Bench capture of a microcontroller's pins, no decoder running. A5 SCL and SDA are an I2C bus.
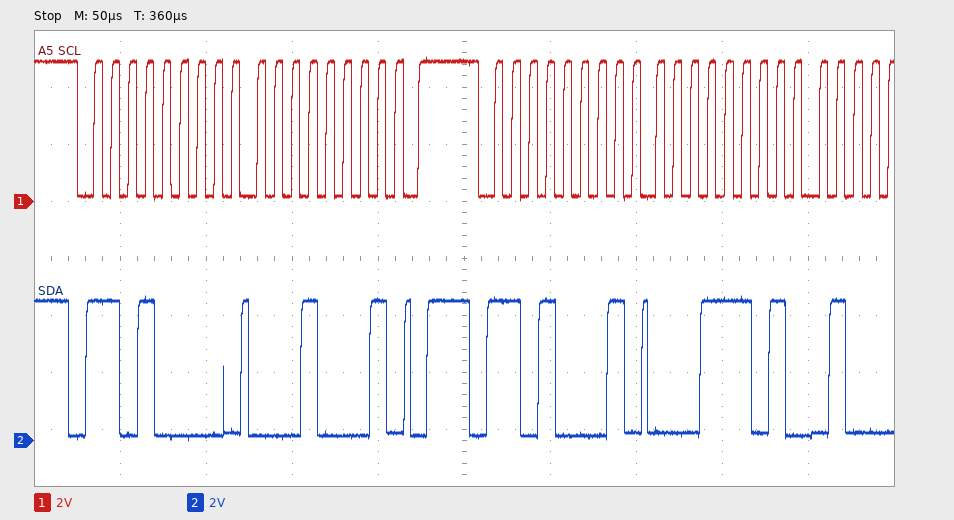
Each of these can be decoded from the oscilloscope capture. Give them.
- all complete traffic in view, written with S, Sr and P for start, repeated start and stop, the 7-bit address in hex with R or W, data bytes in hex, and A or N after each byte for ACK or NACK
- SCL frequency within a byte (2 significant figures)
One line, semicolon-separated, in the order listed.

S 68W A 11 A P S 68R A 1D A; 100 kHz
